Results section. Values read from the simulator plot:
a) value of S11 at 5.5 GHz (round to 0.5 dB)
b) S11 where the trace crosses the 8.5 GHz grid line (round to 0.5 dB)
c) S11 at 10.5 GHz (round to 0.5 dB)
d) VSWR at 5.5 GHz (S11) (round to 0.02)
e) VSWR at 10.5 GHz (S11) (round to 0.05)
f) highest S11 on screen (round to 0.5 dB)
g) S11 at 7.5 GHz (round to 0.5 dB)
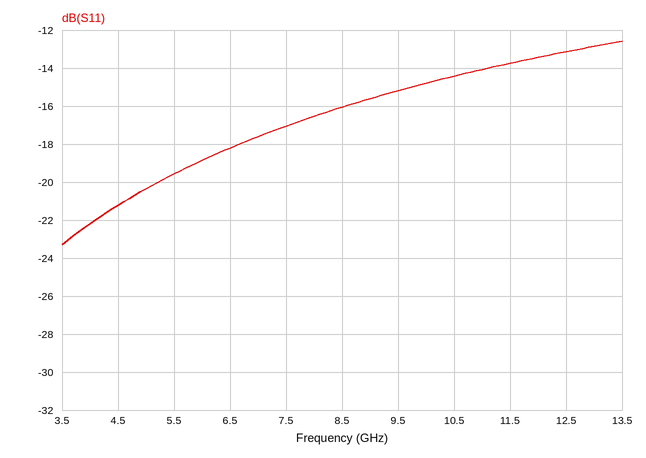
-19.5 dB
-16.0 dB
-14.5 dB
1.24
1.45
-12.5 dB
-17.0 dB
